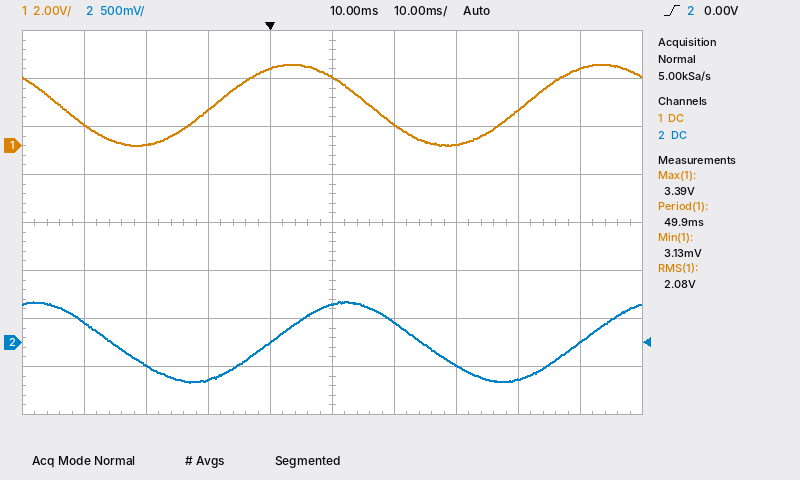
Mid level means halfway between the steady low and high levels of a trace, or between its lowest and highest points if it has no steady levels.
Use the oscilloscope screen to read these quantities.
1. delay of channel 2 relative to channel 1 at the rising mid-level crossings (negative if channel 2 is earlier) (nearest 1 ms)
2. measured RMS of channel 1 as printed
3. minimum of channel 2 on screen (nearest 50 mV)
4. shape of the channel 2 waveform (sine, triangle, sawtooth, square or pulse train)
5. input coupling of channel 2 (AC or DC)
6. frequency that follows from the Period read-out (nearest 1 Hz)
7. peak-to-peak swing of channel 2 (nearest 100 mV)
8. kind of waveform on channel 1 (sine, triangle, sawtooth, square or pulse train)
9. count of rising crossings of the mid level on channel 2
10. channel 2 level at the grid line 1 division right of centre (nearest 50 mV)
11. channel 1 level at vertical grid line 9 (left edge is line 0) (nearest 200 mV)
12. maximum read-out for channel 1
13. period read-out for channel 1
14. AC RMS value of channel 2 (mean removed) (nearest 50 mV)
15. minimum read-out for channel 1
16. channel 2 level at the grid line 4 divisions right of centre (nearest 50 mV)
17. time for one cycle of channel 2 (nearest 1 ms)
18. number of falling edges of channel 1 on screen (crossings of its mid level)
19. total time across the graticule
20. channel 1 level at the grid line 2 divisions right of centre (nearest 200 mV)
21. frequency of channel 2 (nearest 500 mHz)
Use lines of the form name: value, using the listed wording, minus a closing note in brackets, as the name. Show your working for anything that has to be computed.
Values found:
delay of channel 2 relative to channel 1 at the rising mid-level crossings (negative if channel 2 is earlier): +9 ms
measured RMS of channel 1 as printed: 2.08 V
minimum of channel 2 on screen: -400 mV
shape of the channel 2 waveform: sine
input coupling of channel 2: DC
frequency that follows from the Period read-out: 1 / 49.9 ms ≈ 20 Hz
peak-to-peak swing of channel 2: 800 mV
kind of waveform on channel 1: sine
count of rising crossings of the mid level on channel 2: 2
channel 2 level at the grid line 1 division right of centre: 200 mV
channel 1 level at vertical grid line 9 (left edge is line 0): 3.2 V
maximum read-out for channel 1: 3.39 V
period read-out for channel 1: 49.9 ms
AC RMS value of channel 2 (mean removed): 800 mV / (2√2) ≈ 283 mV, so 300 mV to the nearest 50 mV
minimum read-out for channel 1: 3.13 mV
channel 2 level at the grid line 4 divisions right of centre: 0 mV
time for one cycle of channel 2: 50 ms
number of falling edges of channel 1 on screen: 2
total time across the graticule: 100 ms
channel 1 level at the grid line 2 divisions right of centre: 0.0 V
frequency of channel 2: 1 / 50 ms ≈ 20.0 Hz
